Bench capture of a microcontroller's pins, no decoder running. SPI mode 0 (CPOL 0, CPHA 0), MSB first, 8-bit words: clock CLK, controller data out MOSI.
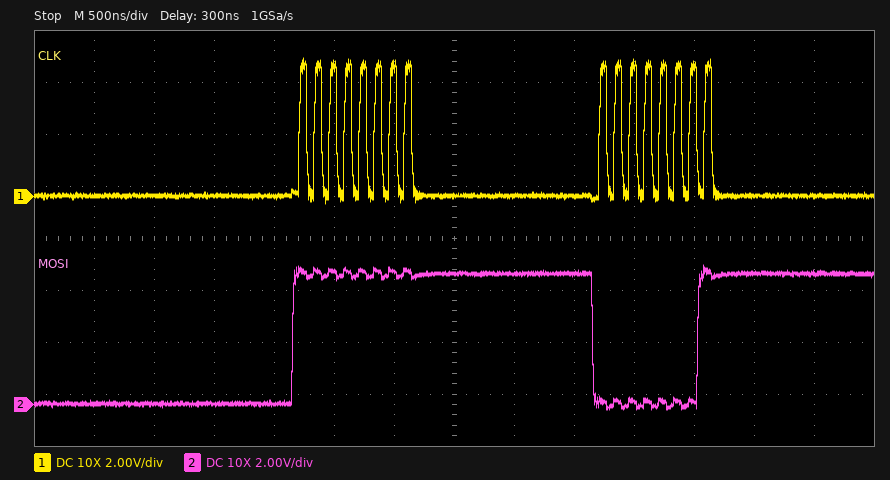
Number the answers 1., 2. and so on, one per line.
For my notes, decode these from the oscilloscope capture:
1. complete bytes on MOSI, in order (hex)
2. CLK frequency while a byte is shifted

1. FF 01
2. 8 MHz
